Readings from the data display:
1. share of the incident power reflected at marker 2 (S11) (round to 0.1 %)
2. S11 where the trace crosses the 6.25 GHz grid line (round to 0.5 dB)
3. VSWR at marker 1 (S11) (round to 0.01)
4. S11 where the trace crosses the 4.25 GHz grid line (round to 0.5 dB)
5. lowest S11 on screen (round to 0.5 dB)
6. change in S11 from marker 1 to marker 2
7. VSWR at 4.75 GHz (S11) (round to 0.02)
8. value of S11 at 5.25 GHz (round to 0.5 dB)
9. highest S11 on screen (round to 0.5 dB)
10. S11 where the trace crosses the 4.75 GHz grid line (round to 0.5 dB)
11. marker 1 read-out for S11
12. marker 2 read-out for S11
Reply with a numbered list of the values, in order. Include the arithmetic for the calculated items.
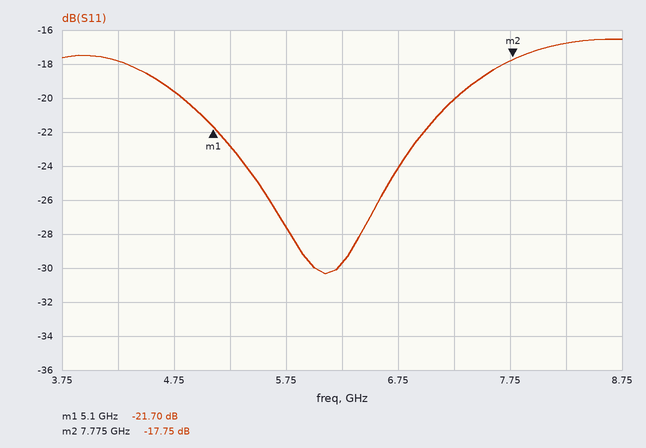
1. 10^(-17.75/10) ≈ 1.7 %
2. -29.5 dB
3. (1 + 0.0822)/(1 − 0.0822) ≈ 1.18
4. -18.0 dB
5. -30.5 dB
6. -17.75 − (-21.7) = 3.95 dB
7. |Γ| = 10^(-19.5/20) = 0.1059; VSWR = (1 + 0.1059)/(1 − 0.1059) ≈ 1.24
8. -23.0 dB
9. -16.5 dB
10. -19.5 dB
11. -21.70 dB
12. -17.75 dB
